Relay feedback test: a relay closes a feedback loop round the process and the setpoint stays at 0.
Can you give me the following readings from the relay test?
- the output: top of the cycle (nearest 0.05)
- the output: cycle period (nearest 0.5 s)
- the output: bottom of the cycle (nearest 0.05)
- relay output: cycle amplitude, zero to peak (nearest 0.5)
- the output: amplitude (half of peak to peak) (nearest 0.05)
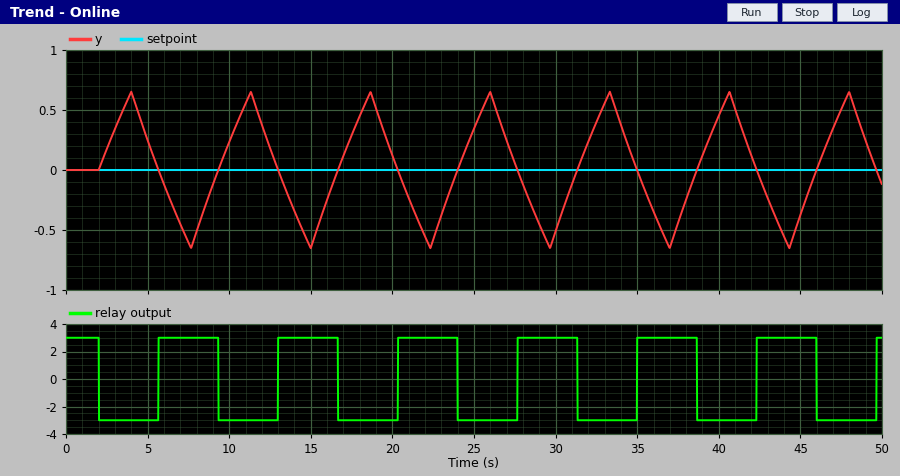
0.65
7.5 s
-0.65
3.0
0.65
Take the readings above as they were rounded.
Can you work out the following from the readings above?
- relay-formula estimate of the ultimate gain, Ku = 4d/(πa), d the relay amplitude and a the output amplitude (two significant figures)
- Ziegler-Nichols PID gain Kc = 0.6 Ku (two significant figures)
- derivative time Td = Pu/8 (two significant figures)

5.9
3.5
0.94 s
